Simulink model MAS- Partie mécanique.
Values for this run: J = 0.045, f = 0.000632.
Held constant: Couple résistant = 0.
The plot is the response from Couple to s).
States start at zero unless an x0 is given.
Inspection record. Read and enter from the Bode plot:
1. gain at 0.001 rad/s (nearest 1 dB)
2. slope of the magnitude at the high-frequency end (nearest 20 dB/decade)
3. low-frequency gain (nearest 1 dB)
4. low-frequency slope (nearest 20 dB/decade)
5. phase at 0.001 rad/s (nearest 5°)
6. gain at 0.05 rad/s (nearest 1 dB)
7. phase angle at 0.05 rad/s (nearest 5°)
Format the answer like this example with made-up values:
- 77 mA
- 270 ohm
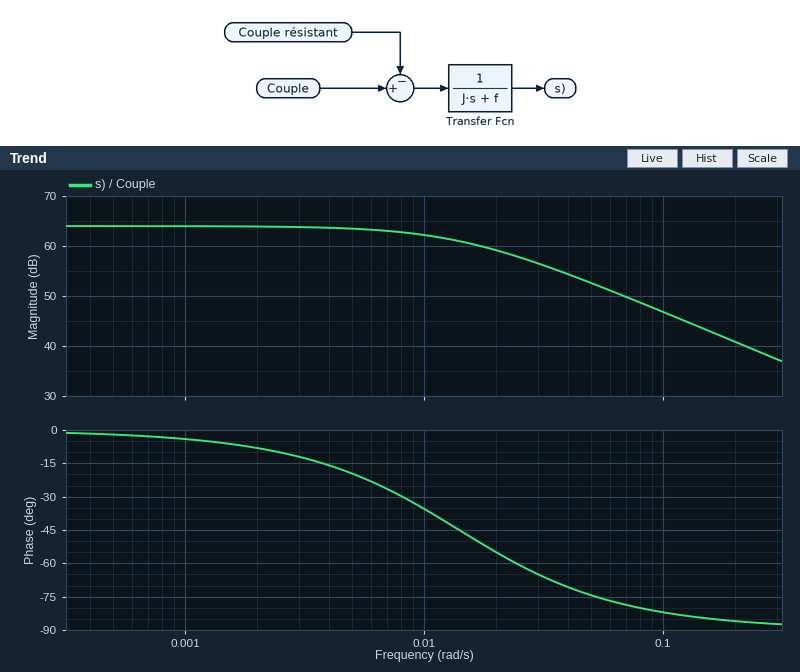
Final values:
- 64 dB
- -20 dB/decade
- 64 dB
- 0 dB/decade
- -5°
- 53 dB
- -75°
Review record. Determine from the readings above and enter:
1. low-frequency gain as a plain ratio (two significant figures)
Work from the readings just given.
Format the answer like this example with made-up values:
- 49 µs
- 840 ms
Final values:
- 1600
